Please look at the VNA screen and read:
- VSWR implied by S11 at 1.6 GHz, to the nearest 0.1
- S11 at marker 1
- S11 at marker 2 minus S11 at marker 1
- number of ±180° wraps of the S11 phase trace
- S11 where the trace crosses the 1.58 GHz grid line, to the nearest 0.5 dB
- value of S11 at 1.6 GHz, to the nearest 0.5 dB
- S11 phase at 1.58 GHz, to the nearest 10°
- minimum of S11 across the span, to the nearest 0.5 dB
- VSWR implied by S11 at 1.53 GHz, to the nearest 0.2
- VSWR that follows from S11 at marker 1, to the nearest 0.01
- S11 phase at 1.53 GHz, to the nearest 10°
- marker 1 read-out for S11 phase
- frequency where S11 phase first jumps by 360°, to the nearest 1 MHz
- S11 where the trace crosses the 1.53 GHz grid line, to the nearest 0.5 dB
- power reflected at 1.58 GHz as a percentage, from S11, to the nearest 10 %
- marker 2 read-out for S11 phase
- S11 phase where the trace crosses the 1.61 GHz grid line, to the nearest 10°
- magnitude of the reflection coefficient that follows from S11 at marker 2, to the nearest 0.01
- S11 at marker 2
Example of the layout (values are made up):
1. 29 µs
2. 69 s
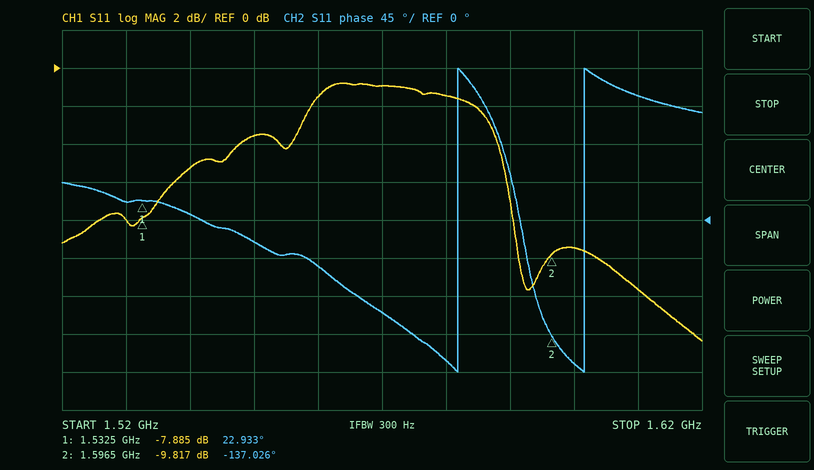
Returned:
1. 2.0
2. -7.885 dB
3. -1.932 dB
4. 2
5. -1.5 dB
6. -9.5 dB
7. -170°
8. -14.5 dB
9. 2.4
10. 2.35
11. 20°
12. 22.933°
13. 1.582 GHz
14. -8.0 dB
15. 70 %
16. -137.026°
17. 150°
18. 0.32
19. -9.817 dB
